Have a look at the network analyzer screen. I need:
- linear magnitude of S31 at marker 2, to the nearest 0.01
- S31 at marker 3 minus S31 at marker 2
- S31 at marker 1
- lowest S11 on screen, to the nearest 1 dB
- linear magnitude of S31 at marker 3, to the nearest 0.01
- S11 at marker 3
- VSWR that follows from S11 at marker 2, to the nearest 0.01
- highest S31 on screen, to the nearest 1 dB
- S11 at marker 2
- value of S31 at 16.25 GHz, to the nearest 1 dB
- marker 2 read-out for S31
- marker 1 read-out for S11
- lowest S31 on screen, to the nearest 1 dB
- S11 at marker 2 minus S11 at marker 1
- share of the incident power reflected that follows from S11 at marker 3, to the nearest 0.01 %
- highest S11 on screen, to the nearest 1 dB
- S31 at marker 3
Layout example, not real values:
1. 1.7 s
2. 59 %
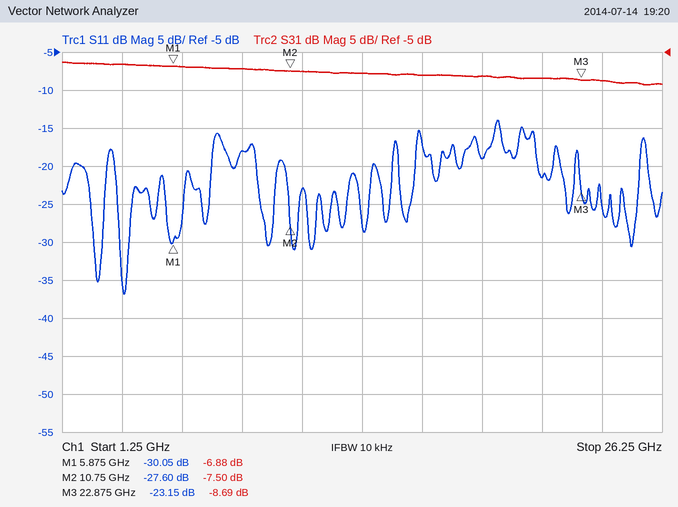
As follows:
1. 0.42
2. -1.19 dB
3. -6.88 dB
4. -37 dB
5. 0.37
6. -23.15 dB
7. 1.09
8. -6 dB
9. -27.60 dB
10. -8 dB
11. -7.50 dB
12. -30.05 dB
13. -9 dB
14. 2.45 dB
15. 0.48 %
16. -14 dB
17. -8.69 dB
